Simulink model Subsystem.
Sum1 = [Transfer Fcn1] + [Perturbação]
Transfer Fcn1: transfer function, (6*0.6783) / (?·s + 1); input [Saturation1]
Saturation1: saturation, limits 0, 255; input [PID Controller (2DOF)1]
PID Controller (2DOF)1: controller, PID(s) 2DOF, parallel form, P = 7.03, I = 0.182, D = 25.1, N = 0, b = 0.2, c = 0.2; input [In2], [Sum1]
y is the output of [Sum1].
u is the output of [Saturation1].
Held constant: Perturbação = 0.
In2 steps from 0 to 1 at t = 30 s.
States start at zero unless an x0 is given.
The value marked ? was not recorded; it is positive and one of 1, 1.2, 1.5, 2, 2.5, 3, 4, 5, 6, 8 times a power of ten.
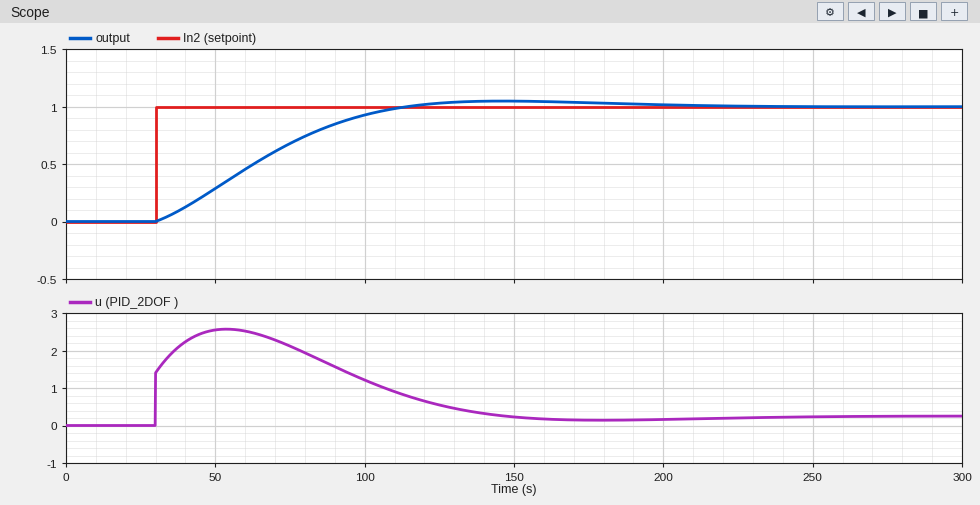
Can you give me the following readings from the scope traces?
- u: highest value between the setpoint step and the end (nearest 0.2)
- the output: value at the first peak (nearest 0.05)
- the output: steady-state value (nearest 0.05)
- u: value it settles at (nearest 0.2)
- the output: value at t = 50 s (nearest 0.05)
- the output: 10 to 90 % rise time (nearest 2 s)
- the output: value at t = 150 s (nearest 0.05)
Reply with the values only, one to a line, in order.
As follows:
2.6
1.05
1.00
0.2
0.30
58 s
1.05
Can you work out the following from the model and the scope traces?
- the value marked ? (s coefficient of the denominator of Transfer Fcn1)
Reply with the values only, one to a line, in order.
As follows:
600
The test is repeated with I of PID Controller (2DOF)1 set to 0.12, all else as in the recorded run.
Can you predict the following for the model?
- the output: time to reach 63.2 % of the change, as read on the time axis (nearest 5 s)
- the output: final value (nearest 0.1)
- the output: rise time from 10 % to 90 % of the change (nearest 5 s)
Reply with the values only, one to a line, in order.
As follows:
85 s
1.0
90 s
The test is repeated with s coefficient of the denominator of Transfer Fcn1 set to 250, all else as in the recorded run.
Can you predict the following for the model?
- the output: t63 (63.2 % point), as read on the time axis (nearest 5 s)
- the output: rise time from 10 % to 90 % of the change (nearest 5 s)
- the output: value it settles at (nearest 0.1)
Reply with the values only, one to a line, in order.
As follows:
65 s
65 s
1.0
